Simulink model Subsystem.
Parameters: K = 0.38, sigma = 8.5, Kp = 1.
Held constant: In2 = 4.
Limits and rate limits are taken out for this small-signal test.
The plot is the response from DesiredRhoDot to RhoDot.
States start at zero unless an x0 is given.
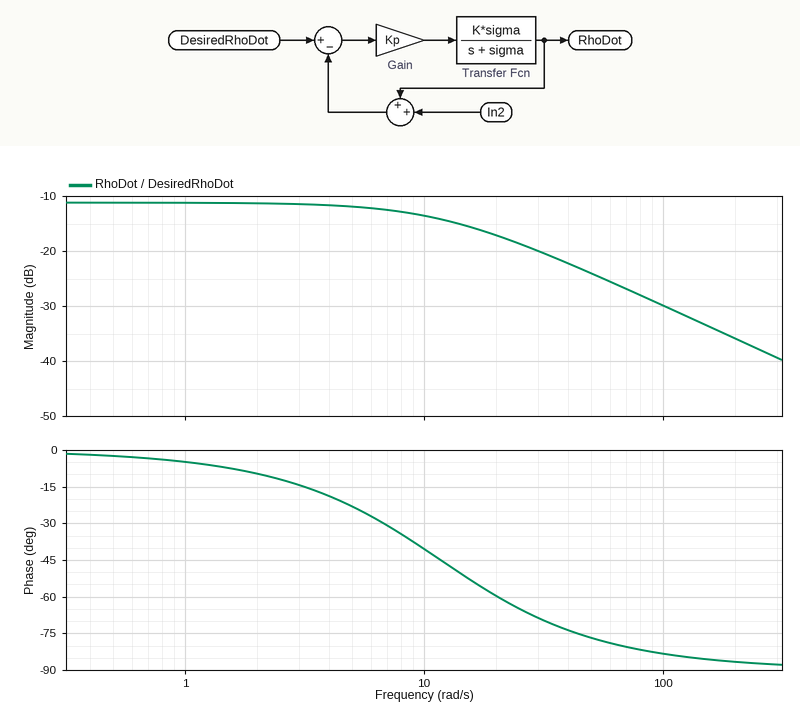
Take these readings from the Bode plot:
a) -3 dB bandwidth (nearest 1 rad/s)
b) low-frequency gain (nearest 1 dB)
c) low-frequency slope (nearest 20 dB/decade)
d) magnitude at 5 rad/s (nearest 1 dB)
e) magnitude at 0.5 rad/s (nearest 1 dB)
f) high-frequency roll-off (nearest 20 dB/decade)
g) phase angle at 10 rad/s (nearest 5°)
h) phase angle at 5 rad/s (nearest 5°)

12 rad/s
-11 dB
0 dB/decade
-12 dB
-11 dB
-20 dB/decade
-40°
-25°
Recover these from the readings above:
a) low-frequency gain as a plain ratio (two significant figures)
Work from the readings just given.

0.28
